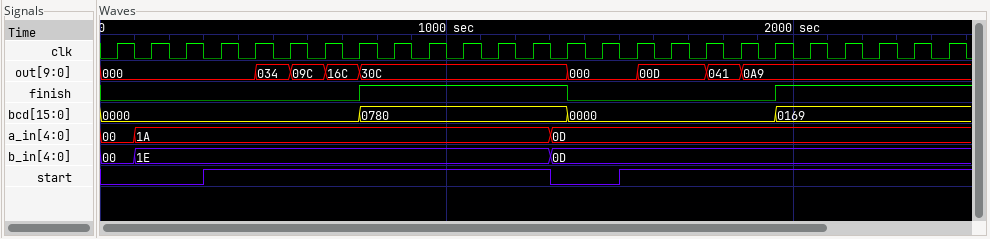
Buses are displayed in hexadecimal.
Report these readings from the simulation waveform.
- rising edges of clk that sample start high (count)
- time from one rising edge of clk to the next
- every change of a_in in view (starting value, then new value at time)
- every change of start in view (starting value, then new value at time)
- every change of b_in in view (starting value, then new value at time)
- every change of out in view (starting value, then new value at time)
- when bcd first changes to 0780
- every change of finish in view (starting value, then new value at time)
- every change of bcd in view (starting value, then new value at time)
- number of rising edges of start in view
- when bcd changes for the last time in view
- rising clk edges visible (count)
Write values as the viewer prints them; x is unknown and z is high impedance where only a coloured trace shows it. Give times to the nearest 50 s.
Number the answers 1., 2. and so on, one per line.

1. 20
2. 100 s
3. 00, 1A at 100 s, 0D at 1300 s
4. 0, 1 at 300 s, 0 at 1300 s, 1 at 1500 s
5. 00, 1E at 100 s, 0D at 1300 s
6. 000, 034 at 450 s, 09C at 550 s, 16C at 650 s, 30C at 750 s, 000 at 1350 s, 00D at 1550 s, 041 at 1750 s, 0A9 at 1850 s
7. 750 s
8. 0, 1 at 750 s, 0 at 1350 s, 1 at 1950 s
9. 0000, 0780 at 750 s, 0000 at 1350 s, 0169 at 1950 s
10. 2
11. 1950 s
12. 25
